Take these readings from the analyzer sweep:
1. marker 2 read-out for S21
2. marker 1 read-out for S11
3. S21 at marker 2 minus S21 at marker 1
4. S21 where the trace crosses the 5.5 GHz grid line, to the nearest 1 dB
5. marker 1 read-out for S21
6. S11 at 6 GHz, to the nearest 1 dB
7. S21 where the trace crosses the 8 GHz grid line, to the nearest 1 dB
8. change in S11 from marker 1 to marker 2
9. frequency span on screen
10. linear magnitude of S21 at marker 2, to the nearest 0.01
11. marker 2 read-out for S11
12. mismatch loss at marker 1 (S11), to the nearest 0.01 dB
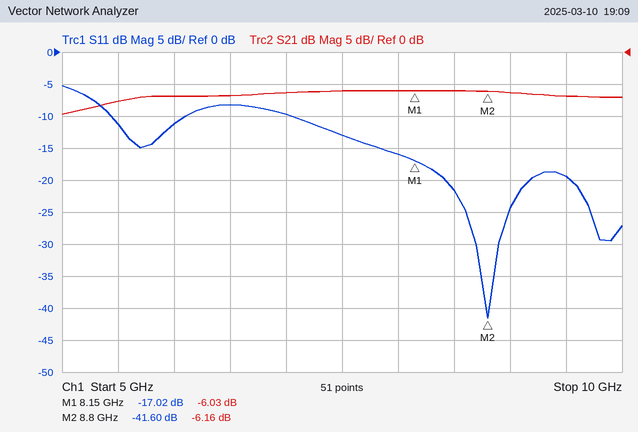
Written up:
-6.16 dB
-17.02 dB
-0.13 dB
-8 dB
-6.03 dB
-11 dB
-6 dB
-24.58 dB
5 GHz
0.49
-41.60 dB
0.09 dB
